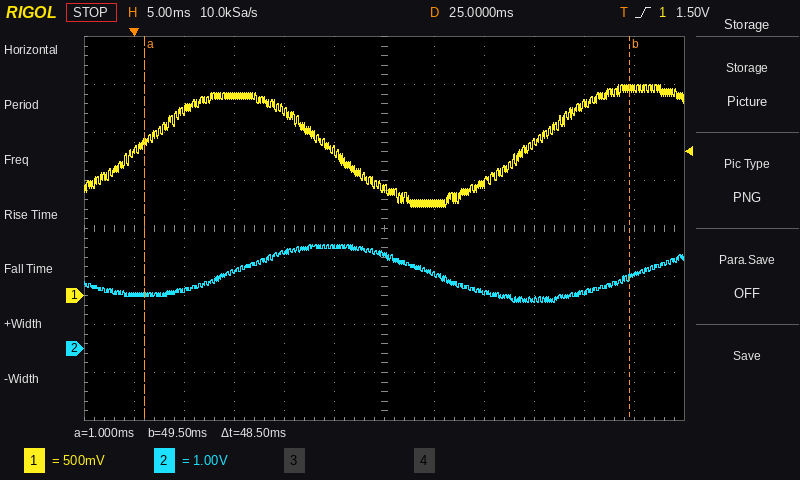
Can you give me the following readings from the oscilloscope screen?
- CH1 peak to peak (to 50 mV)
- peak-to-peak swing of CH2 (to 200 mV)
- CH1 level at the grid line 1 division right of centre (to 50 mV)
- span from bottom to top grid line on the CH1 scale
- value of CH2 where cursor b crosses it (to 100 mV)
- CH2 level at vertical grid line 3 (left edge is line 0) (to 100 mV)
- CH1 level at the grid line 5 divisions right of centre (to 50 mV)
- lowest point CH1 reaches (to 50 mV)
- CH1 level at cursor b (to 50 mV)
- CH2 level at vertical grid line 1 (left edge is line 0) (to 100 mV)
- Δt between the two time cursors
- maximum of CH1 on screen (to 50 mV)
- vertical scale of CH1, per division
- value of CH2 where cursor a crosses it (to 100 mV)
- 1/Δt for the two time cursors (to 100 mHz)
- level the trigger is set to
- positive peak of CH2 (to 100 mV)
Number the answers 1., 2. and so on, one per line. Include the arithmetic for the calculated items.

1. 2.20 V − (900 mV) = 1.30 V
2. 1.2 V
3. 950 mV
4. 4 V
5. 1.5 V
6. 1.6 V
7. 2.15 V
8. 900 mV
9. 2.15 V
10. 1.1 V
11. 48.5 ms
12. 2.20 V
13. 500 mV
14. 1.1 V
15. 1 / 48.5 ms ≈ 20.6 Hz
16. 1.50 V
17. 2.2 V
